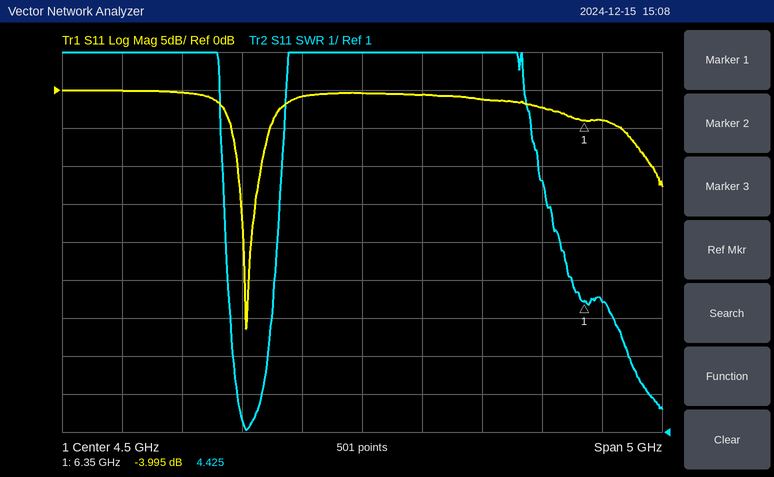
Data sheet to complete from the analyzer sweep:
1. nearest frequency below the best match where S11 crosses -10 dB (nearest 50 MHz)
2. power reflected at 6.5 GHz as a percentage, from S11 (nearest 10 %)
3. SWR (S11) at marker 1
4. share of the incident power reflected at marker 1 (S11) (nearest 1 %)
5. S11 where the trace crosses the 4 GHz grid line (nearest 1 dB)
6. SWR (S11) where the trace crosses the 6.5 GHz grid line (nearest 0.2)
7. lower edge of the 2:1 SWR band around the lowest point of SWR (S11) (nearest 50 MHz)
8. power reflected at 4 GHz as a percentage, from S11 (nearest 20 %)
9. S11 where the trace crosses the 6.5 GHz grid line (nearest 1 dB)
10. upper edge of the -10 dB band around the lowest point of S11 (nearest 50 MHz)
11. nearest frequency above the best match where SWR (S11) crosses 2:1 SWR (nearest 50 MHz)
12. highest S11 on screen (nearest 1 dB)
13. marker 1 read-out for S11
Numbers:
3.45 GHz
40 %
4.425
40 %
-1 dB
4.4
3.45 GHz
80 %
-4 dB
3.65 GHz
3.65 GHz
0 dB
-3.995 dB
